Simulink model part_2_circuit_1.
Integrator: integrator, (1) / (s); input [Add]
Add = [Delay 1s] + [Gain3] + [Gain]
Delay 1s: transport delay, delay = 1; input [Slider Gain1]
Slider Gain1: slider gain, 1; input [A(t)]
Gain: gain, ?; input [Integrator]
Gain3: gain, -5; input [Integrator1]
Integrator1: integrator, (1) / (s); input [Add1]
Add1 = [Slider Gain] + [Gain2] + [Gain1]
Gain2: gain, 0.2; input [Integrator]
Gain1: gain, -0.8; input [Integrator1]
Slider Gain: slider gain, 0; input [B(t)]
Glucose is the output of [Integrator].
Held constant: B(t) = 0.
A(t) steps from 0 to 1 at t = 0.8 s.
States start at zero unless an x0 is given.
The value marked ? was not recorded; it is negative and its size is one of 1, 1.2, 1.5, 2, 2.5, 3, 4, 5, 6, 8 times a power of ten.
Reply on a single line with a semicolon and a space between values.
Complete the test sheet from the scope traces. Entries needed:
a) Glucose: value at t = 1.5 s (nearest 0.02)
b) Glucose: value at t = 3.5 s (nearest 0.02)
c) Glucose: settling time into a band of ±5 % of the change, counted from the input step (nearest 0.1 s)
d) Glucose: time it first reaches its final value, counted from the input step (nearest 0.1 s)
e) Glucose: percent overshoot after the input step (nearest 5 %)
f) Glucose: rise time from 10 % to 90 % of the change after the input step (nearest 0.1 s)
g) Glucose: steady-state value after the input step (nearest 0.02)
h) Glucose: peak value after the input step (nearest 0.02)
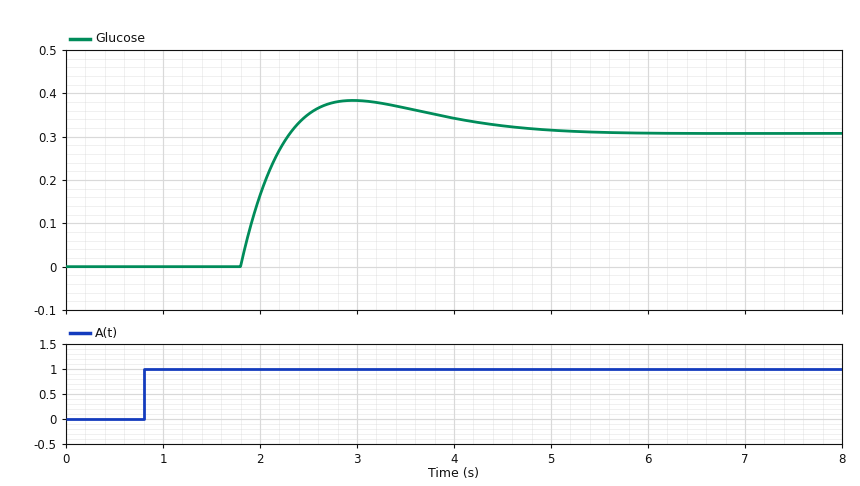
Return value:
0.00; 0.36; 3.8 s; 1.5 s; 25 %; 0.4 s; 0.30; 0.38
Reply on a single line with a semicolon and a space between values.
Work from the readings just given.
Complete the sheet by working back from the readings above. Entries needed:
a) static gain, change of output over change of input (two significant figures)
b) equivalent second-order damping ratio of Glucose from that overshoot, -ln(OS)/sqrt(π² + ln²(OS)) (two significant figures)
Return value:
0.30; 0.40
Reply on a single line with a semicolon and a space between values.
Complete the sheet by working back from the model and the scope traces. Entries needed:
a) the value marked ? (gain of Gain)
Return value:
-2
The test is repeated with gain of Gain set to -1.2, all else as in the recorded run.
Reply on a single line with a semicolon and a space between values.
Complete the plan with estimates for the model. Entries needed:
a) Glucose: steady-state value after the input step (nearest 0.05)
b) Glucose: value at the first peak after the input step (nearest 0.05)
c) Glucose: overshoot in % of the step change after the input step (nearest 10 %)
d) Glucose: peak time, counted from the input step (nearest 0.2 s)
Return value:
0.40; 0.55; 30 %; 2.4 s
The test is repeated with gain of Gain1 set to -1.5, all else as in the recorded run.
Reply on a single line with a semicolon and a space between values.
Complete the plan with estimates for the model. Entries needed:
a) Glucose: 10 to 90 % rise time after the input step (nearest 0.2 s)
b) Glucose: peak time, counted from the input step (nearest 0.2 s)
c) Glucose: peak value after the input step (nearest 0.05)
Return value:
0.6 s; 2.4 s; 0.40
